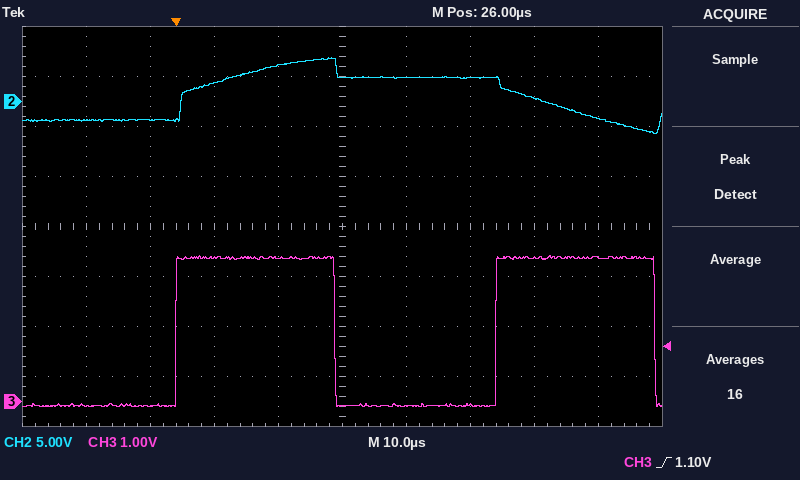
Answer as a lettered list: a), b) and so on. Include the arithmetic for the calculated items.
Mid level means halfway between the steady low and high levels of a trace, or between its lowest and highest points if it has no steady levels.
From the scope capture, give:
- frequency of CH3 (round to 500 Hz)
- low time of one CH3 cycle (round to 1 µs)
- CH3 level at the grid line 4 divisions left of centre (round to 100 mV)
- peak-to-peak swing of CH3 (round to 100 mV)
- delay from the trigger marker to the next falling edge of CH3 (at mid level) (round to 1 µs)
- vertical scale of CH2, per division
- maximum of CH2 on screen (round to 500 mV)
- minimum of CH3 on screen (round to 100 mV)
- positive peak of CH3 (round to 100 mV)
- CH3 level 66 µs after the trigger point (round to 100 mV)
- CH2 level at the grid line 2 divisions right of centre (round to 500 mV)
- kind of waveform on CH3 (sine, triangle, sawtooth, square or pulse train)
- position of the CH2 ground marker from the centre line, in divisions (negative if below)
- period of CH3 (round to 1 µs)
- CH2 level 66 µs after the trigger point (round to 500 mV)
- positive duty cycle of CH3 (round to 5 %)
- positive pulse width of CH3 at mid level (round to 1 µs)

a) 1 / 50 µs ≈ 20.0 kHz
b) 25 µs
c) -100 mV
d) 2.9 V − (-100 mV) = 3.0 V
e) 25 µs
f) 5 V
g) 4.5 V
h) -100 mV
i) 2.9 V
j) 2.9 V
k) 2.5 V
l) square
m) +2.5 div
n) 50 µs
o) -1.5 V
p) 25 µs / 50 µs ≈ 50 %
q) 25 µs
